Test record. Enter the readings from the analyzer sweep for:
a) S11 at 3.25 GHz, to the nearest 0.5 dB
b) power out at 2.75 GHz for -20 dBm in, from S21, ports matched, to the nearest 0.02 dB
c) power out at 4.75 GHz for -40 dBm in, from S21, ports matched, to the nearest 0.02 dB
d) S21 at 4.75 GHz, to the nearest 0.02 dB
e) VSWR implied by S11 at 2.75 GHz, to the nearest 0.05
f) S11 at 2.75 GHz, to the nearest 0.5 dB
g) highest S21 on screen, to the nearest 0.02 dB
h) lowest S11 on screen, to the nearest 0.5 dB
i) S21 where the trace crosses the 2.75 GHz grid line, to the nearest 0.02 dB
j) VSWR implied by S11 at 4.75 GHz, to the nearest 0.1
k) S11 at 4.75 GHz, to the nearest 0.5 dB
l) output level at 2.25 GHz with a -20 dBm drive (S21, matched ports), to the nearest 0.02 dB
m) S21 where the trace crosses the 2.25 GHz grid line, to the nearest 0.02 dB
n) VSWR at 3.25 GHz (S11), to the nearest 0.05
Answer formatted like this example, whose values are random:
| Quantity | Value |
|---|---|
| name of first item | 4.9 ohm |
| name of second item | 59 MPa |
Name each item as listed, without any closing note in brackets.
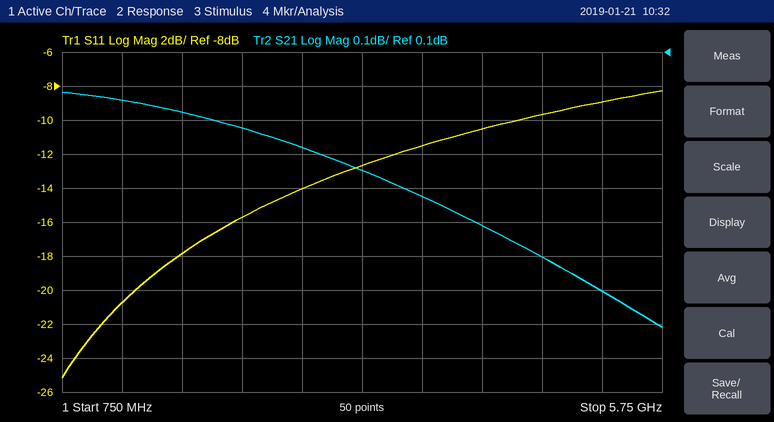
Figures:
| Quantity | Value |
|---|---|
| S11 at 3.25 GHz, to the nearest 0.5 dB | -12.5 dB |
| power out at 2.75 GHz for -20 dBm in, from S21, ports matched, to the nearest 0.02 dB | -20.18 dBm |
| power out at 4.75 GHz for -40 dBm in, from S21, ports matched, to the nearest 0.02 dB | -40.50 dBm |
| S21 at 4.75 GHz, to the nearest 0.02 dB | -0.50 dB |
| VSWR implied by S11 at 2.75 GHz, to the nearest 0.05 | 1.50 |
| S11 at 2.75 GHz, to the nearest 0.5 dB | -14.0 dB |
| highest S21 on screen, to the nearest 0.02 dB | -0.02 dB |
| lowest S11 on screen, to the nearest 0.5 dB | -25.0 dB |
| S21 where the trace crosses the 2.75 GHz grid line, to the nearest 0.02 dB | -0.18 dB |
| VSWR implied by S11 at 4.75 GHz, to the nearest 0.1 | 2.0 |
| S11 at 4.75 GHz, to the nearest 0.5 dB | -9.5 dB |
| output level at 2.25 GHz with a -20 dBm drive (S21, matched ports), to the nearest 0.02 dB | -20.12 dBm |
| S21 where the trace crosses the 2.25 GHz grid line, to the nearest 0.02 dB | -0.12 dB |
| VSWR at 3.25 GHz (S11), to the nearest 0.05 | 1.60 |
